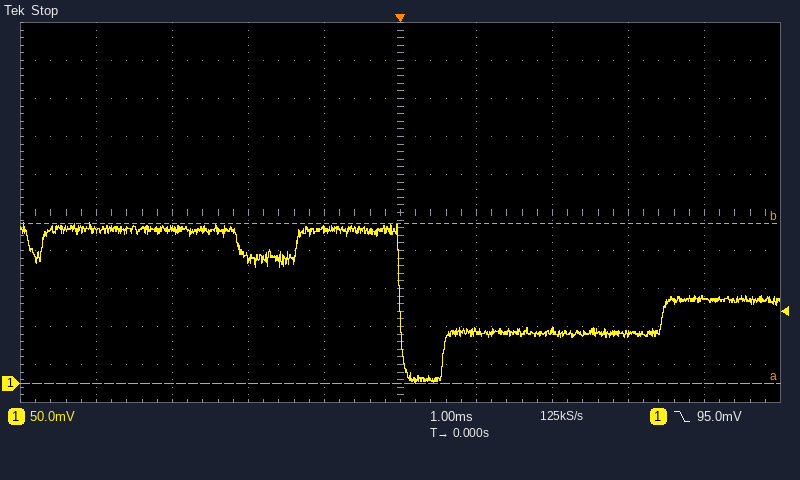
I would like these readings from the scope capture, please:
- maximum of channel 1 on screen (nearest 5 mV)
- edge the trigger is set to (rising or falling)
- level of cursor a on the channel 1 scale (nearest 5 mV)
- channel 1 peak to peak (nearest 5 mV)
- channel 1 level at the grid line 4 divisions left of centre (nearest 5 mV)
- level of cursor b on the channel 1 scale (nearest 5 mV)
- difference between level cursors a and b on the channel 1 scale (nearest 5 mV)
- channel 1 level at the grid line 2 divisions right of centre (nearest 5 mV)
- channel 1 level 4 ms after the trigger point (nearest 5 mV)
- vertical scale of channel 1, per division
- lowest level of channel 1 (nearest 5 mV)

210 mV
falling
0 mV
210 mV
200 mV
210 mV
210 mV
70 mV
110 mV
50 mV
0 mV
